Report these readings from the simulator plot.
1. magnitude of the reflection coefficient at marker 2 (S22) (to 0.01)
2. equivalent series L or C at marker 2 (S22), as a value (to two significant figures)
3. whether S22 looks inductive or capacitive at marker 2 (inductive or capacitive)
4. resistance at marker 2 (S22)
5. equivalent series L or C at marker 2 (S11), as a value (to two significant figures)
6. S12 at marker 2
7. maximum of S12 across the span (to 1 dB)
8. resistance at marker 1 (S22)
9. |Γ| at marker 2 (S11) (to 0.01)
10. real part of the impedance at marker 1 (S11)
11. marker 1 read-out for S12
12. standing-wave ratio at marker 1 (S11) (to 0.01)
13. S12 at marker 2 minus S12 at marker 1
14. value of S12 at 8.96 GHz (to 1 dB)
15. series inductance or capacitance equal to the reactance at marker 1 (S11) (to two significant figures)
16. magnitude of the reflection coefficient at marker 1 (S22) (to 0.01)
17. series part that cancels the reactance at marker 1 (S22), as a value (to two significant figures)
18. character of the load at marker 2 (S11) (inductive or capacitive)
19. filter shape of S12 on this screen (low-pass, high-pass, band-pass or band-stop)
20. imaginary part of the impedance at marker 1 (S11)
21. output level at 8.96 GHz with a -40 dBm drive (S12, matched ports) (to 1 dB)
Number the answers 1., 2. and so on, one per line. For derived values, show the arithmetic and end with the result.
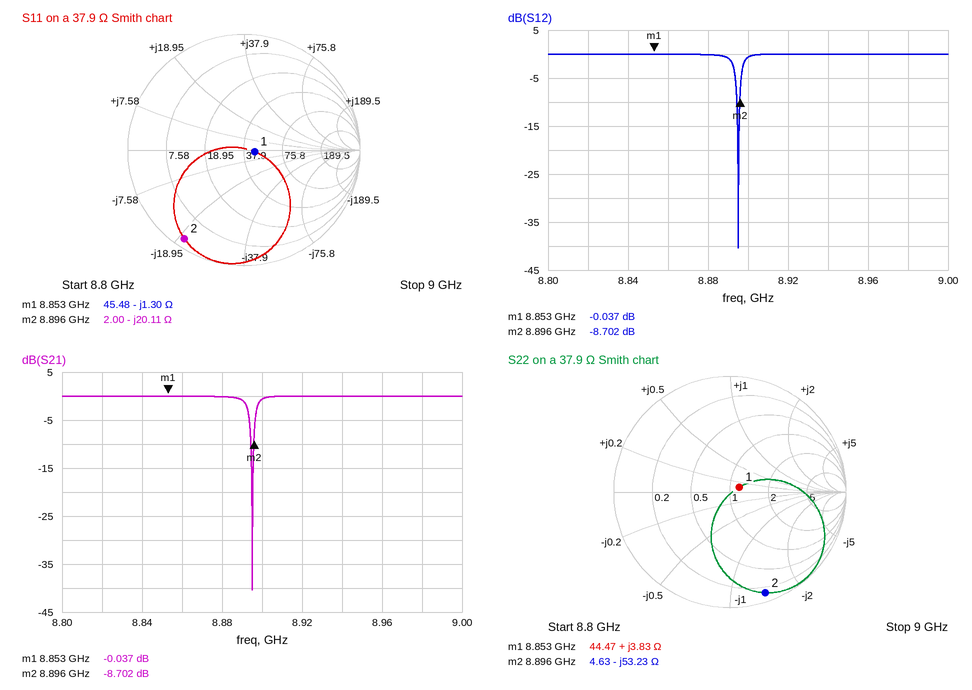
1. 0.92
2. C = 1/(2π × 8.896 GHz × 53.23 Ω) ≈ 336 fF, so 340 fF to two significant figures
3. capacitive
4. 4.63 Ω
5. C = 1/(2π × 8.896 GHz × 20.11 Ω) ≈ 890 fF
6. -8.702 dB
7. 0 dB
8. 44.47 Ω
9. 0.92
10. 45.48 Ω
11. -0.037 dB
12. 1.20
13. -8.702 − (-0.037) = -8.665 dB
14. 0 dB
15. C = 1/(2π × 8.853 GHz × 1.3 Ω) ≈ 14 pF
16. 0.09
17. C = 1/(2π × 8.853 GHz × 3.83 Ω) ≈ 4.7 pF
18. capacitive
19. band-stop
20. -1.30 Ω
21. -40 dBm + (0 dB) = -40 dBm
